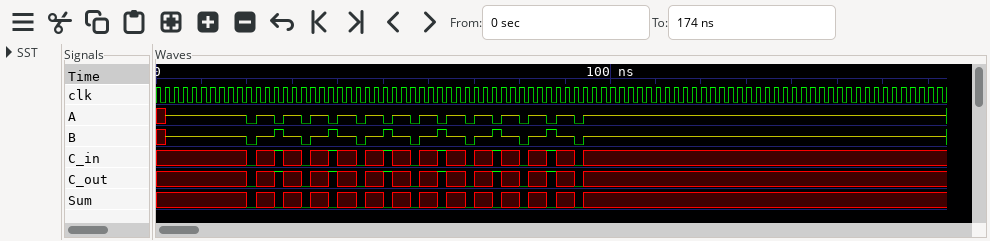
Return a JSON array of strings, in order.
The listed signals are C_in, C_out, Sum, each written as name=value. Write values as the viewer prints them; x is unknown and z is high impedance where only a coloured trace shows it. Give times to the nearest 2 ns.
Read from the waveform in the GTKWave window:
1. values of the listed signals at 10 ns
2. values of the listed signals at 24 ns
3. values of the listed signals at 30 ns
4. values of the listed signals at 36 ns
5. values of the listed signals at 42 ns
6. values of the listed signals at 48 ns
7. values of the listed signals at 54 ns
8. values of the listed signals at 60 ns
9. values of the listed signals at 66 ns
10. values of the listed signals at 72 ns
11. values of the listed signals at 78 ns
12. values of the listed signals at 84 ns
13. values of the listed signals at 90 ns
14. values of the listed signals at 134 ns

["C_in=x, C_out=x, Sum=x", "C_in=x, C_out=x, Sum=x", "C_in=x, C_out=x, Sum=x", "C_in=x, C_out=x, Sum=x", "C_in=x, C_out=x, Sum=x", "C_in=x, C_out=x, Sum=x", "C_in=x, C_out=x, Sum=x", "C_in=x, C_out=x, Sum=x", "C_in=x, C_out=x, Sum=x", "C_in=x, C_out=x, Sum=x", "C_in=x, C_out=x, Sum=x", "C_in=x, C_out=x, Sum=x", "C_in=x, C_out=x, Sum=x", "C_in=x, C_out=x, Sum=x"]
